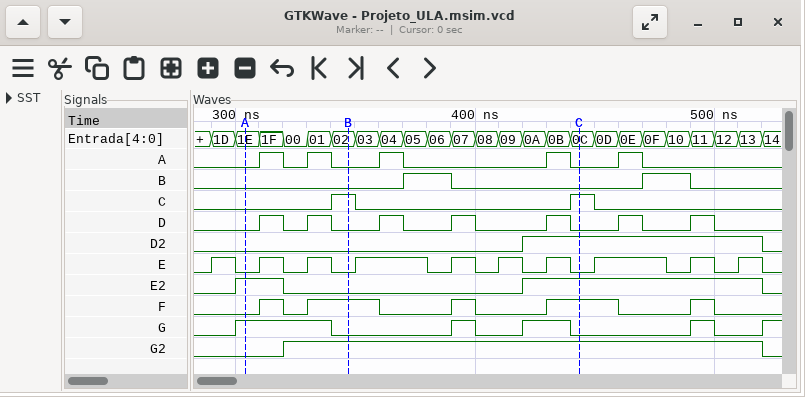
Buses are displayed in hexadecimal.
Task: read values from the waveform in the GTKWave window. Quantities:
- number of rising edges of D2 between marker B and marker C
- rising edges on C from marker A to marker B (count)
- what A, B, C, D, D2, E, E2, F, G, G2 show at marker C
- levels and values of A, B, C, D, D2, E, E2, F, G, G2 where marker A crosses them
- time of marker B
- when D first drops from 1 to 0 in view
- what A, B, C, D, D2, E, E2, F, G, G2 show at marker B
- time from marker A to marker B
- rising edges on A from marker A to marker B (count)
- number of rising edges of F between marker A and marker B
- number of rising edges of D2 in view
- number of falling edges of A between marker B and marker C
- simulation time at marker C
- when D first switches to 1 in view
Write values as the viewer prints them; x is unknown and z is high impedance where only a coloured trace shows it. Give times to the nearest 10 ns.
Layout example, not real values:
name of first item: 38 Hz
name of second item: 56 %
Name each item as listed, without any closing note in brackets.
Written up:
number of rising edges of D2 between marker B and marker C: 1
rising edges on C from marker A to marker B: 1
what A, B, C, D, D2, E, E2, F, G, G2 show at marker C: A=0, B=0, C=1, D=0, D2=1, E=0, E2=1, F=1, G=0, G2=1
levels and values of A, B, C, D, D2, E, E2, F, G, G2 where marker A crosses them: A=0, B=0, C=0, D=0, D2=0, E=0, E2=1, F=0, G=1, G2=0
time of marker B: 350 ns
when D first drops from 1 to 0 in view: 320 ns
what A, B, C, D, D2, E, E2, F, G, G2 show at marker B: A=0, B=0, C=1, D=0, D2=0, E=0, E2=0, F=1, G=0, G2=1
time from marker A to marker B: 40 ns
rising edges on A from marker A to marker B: 2
number of rising edges of F between marker A and marker B: 2
number of rising edges of D2 in view: 1
number of falling edges of A between marker B and marker C: 2
simulation time at marker C: 440 ns
when D first switches to 1 in view: 310 ns
